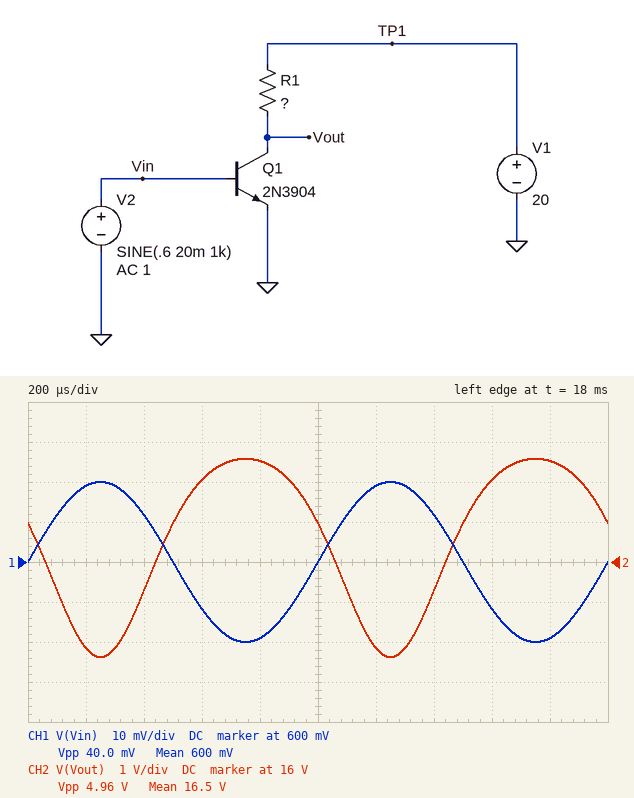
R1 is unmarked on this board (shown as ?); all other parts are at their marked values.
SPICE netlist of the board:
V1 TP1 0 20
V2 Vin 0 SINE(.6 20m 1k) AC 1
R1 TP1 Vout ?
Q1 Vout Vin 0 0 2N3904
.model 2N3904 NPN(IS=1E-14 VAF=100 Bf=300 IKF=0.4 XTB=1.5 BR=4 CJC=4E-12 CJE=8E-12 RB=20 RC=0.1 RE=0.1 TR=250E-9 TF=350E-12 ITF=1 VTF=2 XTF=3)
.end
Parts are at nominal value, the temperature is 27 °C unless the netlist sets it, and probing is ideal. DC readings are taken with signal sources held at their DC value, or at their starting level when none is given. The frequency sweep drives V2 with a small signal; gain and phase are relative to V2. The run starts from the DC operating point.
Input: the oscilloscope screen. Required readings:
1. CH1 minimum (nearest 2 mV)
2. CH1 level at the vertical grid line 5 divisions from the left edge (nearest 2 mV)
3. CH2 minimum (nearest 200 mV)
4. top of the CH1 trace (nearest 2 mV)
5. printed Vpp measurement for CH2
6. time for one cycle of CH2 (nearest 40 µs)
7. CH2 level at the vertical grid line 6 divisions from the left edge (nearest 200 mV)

580 mV
600 mV
13.6 V
620 mV
4.96 V
1.00 ms
13.8 V
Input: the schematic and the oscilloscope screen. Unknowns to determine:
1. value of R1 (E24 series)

22 kΩ
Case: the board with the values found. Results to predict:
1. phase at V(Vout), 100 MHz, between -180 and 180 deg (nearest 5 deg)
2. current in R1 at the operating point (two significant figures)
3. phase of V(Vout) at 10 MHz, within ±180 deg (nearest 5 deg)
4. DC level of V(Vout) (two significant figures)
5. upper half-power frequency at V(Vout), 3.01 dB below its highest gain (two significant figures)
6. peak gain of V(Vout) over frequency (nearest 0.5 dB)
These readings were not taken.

75 deg
140 µA
115 deg
17 V
4.7 MHz
41.0 dB
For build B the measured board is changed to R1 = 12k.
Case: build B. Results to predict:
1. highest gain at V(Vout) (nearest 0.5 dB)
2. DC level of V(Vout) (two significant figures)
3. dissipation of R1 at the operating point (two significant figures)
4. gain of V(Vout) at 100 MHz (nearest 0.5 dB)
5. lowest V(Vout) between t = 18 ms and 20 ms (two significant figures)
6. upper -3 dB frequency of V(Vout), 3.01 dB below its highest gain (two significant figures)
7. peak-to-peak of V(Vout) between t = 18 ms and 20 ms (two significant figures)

36.0 dB
18 V
230 µW
15.0 dB
16 V
8.7 MHz
2.8 V
